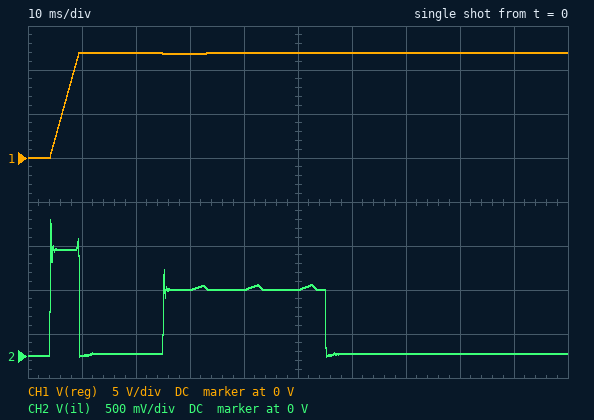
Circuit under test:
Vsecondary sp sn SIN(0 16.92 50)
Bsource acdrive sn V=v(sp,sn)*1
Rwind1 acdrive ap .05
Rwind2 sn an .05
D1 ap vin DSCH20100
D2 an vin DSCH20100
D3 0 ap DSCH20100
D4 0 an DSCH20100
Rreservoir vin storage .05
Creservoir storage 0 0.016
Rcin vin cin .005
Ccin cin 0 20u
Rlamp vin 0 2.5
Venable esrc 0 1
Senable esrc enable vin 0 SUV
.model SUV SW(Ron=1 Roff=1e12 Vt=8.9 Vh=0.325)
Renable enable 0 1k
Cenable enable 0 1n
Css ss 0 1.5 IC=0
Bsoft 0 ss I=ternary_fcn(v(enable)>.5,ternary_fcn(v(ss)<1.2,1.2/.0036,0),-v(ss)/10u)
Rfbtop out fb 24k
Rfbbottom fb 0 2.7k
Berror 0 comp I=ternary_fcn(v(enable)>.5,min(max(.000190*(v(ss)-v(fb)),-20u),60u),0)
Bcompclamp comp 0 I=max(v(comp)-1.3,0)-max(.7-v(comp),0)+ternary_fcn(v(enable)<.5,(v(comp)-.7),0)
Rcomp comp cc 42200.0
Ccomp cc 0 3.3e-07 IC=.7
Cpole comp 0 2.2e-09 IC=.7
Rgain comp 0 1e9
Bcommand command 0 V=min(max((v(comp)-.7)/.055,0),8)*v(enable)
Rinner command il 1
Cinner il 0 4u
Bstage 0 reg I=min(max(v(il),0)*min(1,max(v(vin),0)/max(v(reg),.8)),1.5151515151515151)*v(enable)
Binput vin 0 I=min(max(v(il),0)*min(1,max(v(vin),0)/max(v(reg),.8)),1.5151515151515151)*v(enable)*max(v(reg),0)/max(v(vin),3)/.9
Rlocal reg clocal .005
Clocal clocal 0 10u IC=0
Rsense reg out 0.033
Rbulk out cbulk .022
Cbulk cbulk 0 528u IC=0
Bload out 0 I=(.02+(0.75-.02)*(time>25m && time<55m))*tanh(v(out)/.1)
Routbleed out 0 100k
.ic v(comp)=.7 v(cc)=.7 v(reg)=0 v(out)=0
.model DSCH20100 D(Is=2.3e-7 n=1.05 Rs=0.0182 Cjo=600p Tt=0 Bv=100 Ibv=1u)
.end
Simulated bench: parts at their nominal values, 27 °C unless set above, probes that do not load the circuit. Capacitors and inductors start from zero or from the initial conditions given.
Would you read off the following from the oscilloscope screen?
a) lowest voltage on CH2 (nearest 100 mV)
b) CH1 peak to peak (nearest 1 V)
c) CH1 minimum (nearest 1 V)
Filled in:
0 V
12 V
0 V
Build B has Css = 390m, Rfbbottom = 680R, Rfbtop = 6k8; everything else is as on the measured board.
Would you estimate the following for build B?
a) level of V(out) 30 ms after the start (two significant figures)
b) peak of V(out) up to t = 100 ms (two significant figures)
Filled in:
13 V
14 V
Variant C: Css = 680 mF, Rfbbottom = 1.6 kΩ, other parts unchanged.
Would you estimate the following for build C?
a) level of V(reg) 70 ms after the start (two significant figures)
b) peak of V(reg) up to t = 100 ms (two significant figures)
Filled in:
19 V
20 V
